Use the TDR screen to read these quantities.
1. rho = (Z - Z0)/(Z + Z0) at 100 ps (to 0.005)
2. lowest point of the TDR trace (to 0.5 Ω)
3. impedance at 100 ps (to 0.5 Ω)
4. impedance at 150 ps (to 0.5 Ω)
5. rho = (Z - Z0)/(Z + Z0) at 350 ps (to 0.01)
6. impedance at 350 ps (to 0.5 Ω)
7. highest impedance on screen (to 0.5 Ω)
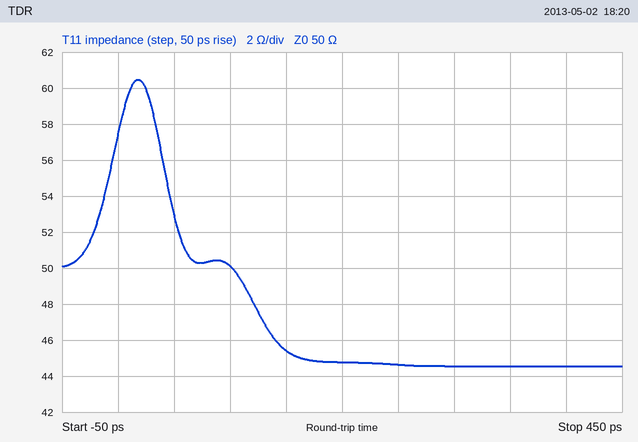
0.000
44.5 Ω
50.0 Ω
45.5 Ω
-0.06
44.5 Ω
60.5 Ω
